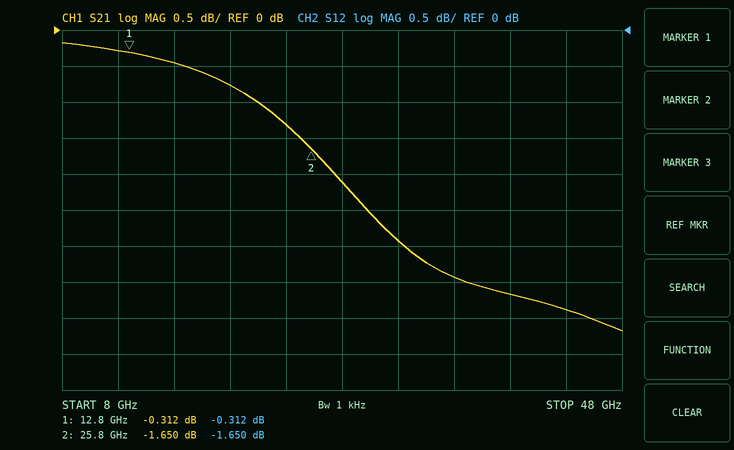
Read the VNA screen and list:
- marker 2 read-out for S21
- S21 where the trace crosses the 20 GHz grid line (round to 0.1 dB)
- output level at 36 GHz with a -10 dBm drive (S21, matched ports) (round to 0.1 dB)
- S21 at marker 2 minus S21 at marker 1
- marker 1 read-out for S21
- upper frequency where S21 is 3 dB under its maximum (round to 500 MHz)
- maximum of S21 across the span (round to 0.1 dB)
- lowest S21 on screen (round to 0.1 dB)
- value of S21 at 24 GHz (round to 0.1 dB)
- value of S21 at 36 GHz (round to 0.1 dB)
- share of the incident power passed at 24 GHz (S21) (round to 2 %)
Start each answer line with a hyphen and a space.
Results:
- -1.650 dB
- -0.8 dB
- -13.4 dBm
- -1.338 dB
- -0.312 dB
- 33.5 GHz
- -0.2 dB
- -4.2 dB
- -1.3 dB
- -3.4 dB
- 74 %
